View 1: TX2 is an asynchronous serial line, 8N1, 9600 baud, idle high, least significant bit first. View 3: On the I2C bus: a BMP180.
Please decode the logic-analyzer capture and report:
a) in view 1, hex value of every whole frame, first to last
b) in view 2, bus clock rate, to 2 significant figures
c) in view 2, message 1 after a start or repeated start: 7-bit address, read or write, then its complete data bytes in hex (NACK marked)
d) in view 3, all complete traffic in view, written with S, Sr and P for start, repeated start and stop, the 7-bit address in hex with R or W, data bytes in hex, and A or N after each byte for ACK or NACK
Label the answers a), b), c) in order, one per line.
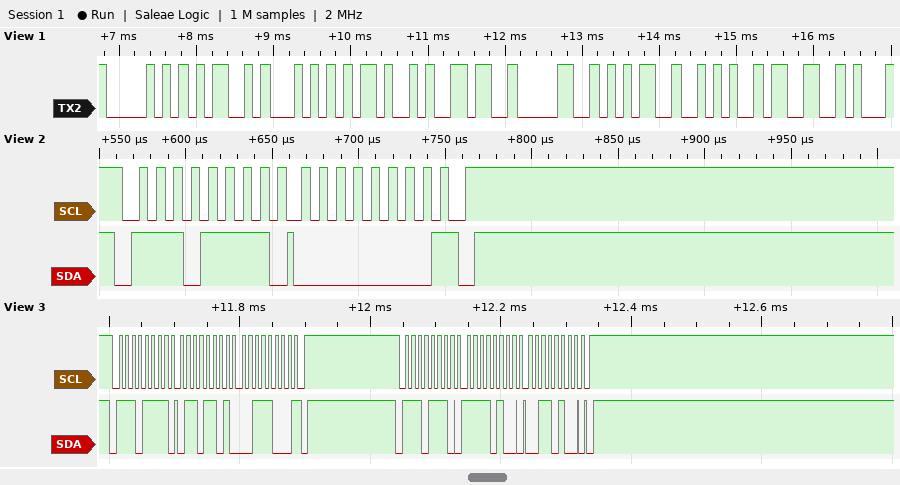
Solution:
a) 0x50 0x4D 0x54 0x4B 0x36 0x30 0x35 0x2A 0x33
b) 100 kHz
c) 0x77 read: 00 NACK
d) S 77R A 6D A 38 N P S 77W A F4 A 34 A P
